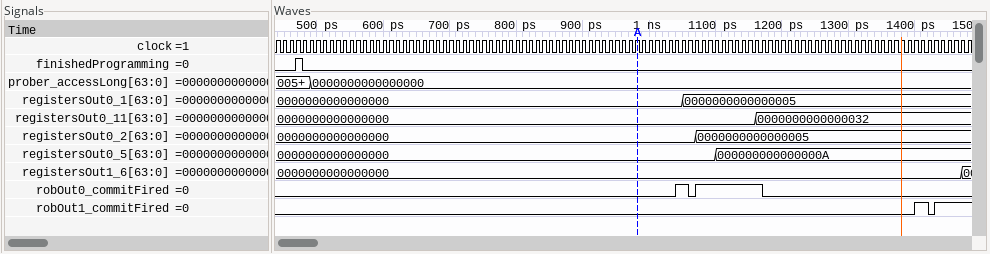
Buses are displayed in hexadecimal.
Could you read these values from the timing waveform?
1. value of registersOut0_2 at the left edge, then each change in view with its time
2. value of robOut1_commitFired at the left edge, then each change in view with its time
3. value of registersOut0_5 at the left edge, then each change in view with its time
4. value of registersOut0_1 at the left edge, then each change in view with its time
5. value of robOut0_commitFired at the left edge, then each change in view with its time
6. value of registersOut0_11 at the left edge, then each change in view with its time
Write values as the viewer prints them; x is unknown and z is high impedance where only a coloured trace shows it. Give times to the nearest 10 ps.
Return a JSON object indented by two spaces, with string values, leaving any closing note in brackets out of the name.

{
  "value of registersOut0_2 at the left edge, then each change in view with its time": "0000000000000000, 0000000000000005 at 1070 ps",
  "value of robOut1_commitFired at the left edge, then each change in view with its time": "0, 1 at 1400 ps, 0 at 1420 ps, 1 at 1430 ps",
  "value of registersOut0_5 at the left edge, then each change in view with its time": "0000000000000000, 000000000000000A at 1100 ps",
  "value of registersOut0_1 at the left edge, then each change in view with its time": "0000000000000000, 0000000000000005 at 1050 ps",
  "value of robOut0_commitFired at the left edge, then each change in view with its time": "0, 1 at 1040 ps, 0 at 1060 ps, 1 at 1070 ps, 0 at 1170 ps",
  "value of registersOut0_11 at the left edge, then each change in view with its time": "0000000000000000, 0000000000000032 at 1160 ps"
}
